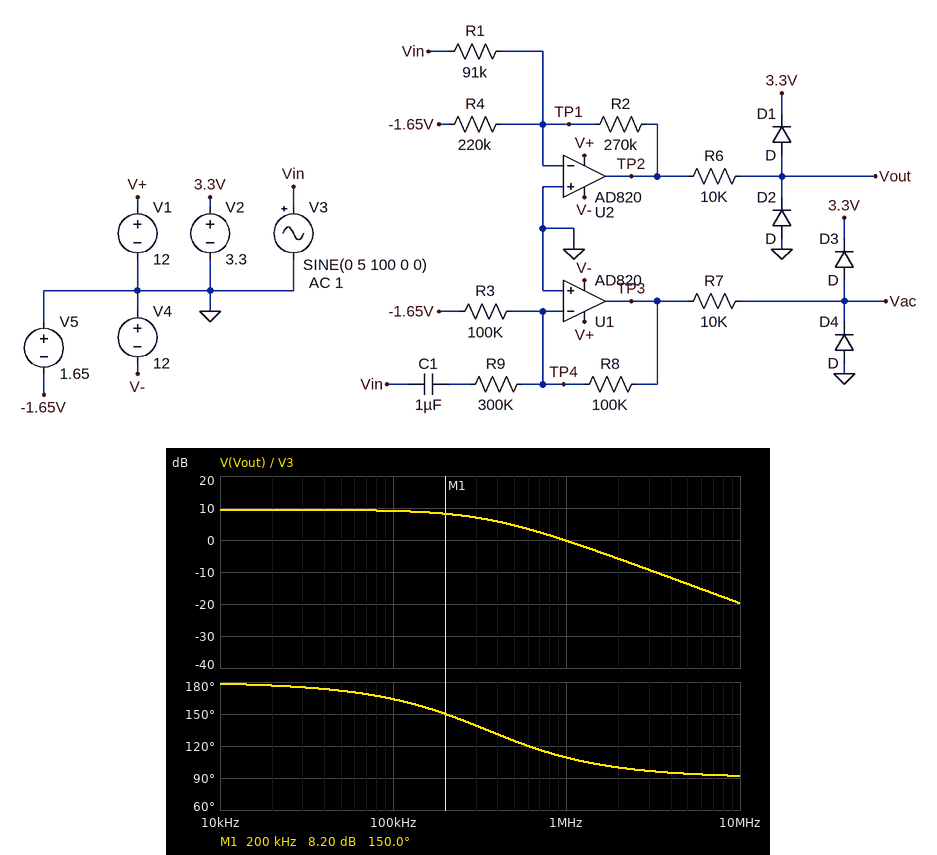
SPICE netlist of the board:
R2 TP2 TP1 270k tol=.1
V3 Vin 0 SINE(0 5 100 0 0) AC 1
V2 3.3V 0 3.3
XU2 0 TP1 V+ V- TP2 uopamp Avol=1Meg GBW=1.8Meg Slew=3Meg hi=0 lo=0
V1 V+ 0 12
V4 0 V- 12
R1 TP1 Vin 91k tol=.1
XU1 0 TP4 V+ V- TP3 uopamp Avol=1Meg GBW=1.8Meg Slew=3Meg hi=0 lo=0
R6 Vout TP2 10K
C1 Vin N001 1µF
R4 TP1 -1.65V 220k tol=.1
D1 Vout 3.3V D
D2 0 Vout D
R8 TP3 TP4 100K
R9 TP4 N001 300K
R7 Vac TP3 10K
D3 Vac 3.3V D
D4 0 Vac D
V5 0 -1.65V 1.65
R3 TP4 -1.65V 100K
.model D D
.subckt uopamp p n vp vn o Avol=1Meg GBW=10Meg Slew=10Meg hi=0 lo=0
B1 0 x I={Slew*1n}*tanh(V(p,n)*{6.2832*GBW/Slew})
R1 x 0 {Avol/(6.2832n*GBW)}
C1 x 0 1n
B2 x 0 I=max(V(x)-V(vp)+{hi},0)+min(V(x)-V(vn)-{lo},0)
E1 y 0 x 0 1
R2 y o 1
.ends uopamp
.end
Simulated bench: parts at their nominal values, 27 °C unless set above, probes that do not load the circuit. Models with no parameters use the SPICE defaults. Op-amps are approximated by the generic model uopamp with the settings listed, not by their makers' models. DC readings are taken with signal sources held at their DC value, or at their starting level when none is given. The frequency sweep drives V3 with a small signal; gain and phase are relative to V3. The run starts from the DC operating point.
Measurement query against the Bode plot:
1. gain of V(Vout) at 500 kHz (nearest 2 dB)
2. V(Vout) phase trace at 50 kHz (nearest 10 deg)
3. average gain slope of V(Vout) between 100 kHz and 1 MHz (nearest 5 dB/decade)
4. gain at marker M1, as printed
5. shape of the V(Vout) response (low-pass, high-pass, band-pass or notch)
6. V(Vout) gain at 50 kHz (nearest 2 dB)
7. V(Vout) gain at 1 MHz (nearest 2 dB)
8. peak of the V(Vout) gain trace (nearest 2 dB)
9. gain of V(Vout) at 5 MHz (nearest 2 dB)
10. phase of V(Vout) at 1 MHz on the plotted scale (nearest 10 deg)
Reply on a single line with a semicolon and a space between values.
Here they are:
4 dB; 170 deg; -10 dB/decade; 8.20 dB; low-pass; 10 dB; 0 dB; 10 dB; -14 dB; 110 deg
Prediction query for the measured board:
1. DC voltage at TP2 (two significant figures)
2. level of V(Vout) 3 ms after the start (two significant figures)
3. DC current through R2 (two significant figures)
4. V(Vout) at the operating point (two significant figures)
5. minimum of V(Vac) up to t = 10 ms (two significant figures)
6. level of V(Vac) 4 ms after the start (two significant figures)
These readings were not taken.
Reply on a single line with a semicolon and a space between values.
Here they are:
2.0 V; -660 mV; 7.5 µA; 2.0 V; -7.9 mV; 690 mV
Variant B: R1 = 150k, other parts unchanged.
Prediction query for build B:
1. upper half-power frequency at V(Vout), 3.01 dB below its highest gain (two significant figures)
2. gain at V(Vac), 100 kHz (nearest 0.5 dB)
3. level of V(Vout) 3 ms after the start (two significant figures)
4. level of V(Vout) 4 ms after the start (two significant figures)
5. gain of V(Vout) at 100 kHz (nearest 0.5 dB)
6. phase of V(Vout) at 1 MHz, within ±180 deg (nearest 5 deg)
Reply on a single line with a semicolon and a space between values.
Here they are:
450 kHz; -9.5 dB; -640 mV; -620 mV; 5.0 dB; 115 deg
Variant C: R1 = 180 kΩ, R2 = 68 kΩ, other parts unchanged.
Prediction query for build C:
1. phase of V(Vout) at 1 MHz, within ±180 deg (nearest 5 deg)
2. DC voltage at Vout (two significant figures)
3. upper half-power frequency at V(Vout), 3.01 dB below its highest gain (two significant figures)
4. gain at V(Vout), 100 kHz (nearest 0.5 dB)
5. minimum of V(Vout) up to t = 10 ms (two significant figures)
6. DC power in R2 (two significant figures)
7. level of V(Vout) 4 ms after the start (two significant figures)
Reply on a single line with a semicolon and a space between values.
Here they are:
135 deg; 510 mV; 1.1 MHz; -8.5 dB; -590 mV; 3.8 µW; -530 mV
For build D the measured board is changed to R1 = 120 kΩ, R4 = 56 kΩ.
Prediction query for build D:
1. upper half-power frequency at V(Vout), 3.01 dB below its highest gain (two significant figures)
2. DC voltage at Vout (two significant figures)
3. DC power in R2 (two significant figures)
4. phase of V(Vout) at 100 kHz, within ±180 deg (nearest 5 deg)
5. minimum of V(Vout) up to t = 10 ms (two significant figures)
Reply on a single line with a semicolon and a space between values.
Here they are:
220 kHz; 3.9 V; 230 µW; 155 deg; -620 mV
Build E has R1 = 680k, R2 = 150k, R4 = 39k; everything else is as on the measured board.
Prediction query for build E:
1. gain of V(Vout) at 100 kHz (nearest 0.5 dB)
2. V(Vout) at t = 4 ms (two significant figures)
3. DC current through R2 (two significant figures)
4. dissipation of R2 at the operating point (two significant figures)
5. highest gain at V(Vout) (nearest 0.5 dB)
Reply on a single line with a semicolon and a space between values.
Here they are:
-53.0 dB; 3.9 V; 42 µA; 270 µW; -52.5 dB
